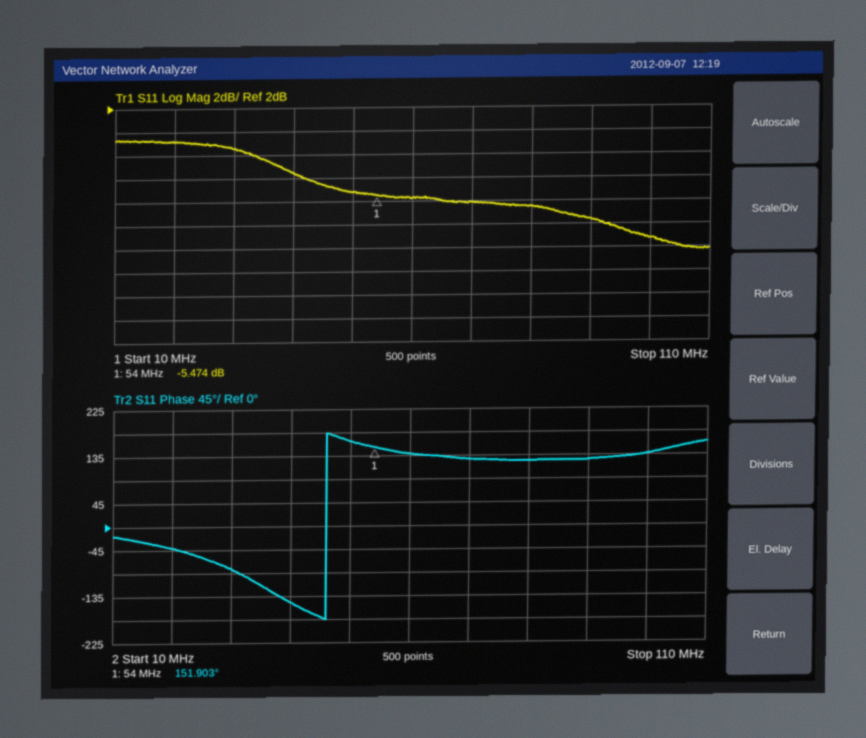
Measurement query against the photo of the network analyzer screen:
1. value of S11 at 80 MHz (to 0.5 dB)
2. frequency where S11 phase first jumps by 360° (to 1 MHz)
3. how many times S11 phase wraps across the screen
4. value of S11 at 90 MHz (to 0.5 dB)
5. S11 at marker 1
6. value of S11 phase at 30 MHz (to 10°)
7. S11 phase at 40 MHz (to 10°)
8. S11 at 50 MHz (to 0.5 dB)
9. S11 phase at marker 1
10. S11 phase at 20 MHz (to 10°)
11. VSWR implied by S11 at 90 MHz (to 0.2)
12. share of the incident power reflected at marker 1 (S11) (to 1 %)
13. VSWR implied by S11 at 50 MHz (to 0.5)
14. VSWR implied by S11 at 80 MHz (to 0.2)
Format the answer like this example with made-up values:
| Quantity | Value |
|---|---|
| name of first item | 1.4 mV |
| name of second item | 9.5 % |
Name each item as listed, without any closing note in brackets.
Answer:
| Quantity | Value |
|---|---|
| value of S11 at 80 MHz | -6.5 dB |
| frequency where S11 phase first jumps by 360° | 46 MHz |
| how many times S11 phase wraps across the screen | 1 |
| value of S11 at 90 MHz | -7.5 dB |
| S11 at marker 1 | -5.474 dB |
| value of S11 phase at 30 MHz | -80° |
| S11 phase at 40 MHz | -150° |
| S11 at 50 MHz | -5.0 dB |
| S11 phase at marker 1 | 151.903° |
| S11 phase at 20 MHz | -40° |
| VSWR implied by S11 at 90 MHz | 2.4 |
| share of the incident power reflected at marker 1 (S11) | 28 % |
| VSWR implied by S11 at 50 MHz | 3.5 |
| VSWR implied by S11 at 80 MHz | 2.8 |
